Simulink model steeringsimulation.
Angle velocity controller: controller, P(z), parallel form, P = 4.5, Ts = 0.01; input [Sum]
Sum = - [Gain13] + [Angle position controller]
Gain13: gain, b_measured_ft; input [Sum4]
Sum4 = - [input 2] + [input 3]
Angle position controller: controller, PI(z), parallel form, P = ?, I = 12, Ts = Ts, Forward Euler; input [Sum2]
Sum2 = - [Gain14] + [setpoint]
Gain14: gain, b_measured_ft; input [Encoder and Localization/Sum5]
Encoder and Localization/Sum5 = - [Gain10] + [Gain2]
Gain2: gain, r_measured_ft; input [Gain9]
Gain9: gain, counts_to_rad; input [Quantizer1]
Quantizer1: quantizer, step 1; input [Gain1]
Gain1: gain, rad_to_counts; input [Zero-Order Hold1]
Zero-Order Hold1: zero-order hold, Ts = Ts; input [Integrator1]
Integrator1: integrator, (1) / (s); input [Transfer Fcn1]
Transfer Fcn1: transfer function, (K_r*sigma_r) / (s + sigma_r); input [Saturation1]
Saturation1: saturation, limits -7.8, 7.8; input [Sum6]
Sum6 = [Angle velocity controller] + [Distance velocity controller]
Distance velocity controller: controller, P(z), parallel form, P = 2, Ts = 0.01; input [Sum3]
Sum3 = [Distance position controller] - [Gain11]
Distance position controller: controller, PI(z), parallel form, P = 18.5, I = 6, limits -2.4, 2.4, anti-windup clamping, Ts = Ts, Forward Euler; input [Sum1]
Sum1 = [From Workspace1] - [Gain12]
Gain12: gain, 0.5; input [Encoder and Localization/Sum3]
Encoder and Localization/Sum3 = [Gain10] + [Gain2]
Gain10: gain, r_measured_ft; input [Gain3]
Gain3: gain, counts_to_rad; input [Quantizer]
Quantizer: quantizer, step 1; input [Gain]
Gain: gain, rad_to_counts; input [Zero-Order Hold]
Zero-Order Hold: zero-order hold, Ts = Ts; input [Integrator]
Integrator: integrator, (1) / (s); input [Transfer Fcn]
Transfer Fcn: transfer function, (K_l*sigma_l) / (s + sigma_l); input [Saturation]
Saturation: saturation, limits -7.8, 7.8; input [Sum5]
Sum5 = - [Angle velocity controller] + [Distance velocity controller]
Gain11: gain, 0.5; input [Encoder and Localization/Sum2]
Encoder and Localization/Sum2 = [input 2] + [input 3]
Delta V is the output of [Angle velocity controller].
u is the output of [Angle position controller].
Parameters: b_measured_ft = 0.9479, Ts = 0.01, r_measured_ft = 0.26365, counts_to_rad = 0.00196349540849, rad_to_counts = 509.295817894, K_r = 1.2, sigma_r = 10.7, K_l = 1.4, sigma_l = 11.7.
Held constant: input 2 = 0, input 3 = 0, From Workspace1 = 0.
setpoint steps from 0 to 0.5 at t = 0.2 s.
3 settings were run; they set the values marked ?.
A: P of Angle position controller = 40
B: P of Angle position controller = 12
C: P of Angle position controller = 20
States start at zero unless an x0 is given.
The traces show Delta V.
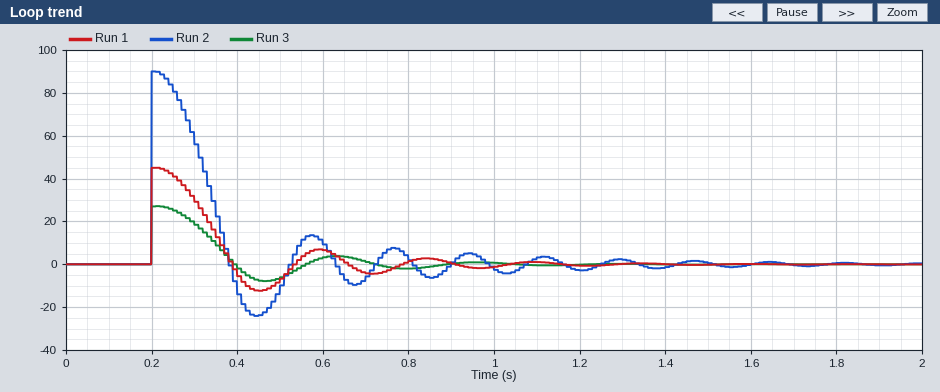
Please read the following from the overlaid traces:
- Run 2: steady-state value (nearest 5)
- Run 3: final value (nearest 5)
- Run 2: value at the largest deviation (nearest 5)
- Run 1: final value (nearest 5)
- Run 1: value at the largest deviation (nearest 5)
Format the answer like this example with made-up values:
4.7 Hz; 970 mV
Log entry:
0; 0; 90; 0; 45
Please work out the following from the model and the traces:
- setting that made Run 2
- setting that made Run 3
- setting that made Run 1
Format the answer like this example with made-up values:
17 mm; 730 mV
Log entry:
A; B; C
